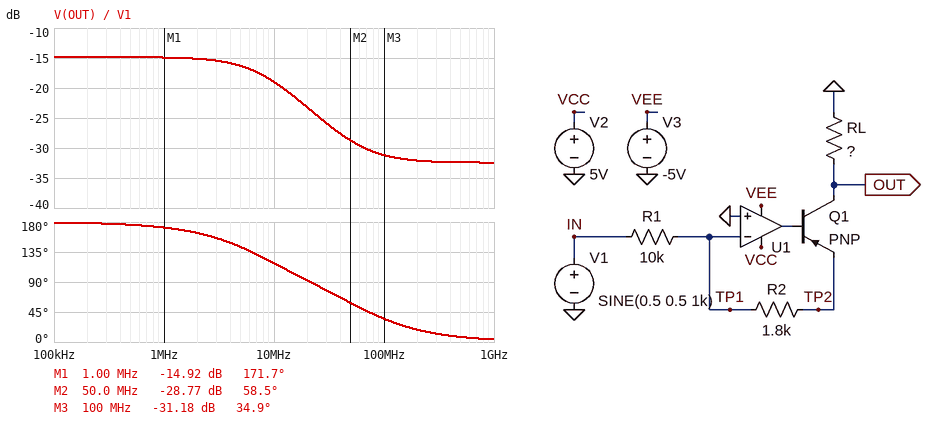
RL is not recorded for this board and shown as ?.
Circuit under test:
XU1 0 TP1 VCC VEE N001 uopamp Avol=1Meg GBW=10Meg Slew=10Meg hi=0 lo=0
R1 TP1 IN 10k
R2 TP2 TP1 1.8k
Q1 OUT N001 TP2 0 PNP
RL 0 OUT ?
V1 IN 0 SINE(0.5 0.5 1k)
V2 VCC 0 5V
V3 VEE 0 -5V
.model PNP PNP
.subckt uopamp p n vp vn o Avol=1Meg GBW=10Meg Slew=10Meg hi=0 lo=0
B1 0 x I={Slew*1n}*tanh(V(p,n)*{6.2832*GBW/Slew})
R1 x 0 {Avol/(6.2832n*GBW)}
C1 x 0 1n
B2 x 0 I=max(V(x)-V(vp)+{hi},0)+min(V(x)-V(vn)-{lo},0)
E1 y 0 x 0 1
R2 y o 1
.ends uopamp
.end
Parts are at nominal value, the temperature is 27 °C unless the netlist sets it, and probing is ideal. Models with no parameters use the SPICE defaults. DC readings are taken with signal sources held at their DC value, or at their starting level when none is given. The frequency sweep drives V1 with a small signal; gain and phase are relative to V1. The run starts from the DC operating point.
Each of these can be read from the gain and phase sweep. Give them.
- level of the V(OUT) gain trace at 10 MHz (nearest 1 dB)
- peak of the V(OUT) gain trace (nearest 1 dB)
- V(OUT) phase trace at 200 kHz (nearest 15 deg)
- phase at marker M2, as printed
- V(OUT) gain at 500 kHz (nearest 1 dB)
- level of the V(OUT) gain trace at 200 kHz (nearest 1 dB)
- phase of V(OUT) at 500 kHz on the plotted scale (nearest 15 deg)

-19 dB
-15 dB
180 deg
58.5 deg
-15 dB
-15 dB
180 deg
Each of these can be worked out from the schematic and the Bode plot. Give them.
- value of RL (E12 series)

3.3 kΩ
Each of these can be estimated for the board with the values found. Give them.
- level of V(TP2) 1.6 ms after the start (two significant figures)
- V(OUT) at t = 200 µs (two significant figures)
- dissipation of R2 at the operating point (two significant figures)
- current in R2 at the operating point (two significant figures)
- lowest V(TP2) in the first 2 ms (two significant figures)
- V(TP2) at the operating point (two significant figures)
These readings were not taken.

-37 mV
-190 mV
4.5 µW
50 µA
-180 mV
-90 mV
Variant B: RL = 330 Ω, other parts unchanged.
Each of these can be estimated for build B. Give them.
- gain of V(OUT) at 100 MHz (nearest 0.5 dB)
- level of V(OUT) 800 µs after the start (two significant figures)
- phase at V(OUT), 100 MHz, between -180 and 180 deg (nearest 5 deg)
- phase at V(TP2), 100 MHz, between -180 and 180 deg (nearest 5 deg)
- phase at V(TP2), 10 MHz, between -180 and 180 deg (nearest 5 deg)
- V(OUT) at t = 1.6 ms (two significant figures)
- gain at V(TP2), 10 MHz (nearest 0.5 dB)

-37.5 dB
-6.8 mV
70 deg
55 deg
120 deg
-40 mV
-19.5 dB
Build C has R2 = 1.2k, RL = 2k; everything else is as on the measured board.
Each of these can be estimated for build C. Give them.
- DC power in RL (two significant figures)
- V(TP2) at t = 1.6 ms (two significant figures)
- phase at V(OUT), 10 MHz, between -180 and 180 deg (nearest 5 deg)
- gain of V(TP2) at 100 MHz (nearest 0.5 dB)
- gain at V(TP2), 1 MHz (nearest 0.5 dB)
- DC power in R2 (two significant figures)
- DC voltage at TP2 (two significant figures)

2.6 µW
-25 mV
115 deg
-30.0 dB
-18.5 dB
3.0 µW
-60 mV
